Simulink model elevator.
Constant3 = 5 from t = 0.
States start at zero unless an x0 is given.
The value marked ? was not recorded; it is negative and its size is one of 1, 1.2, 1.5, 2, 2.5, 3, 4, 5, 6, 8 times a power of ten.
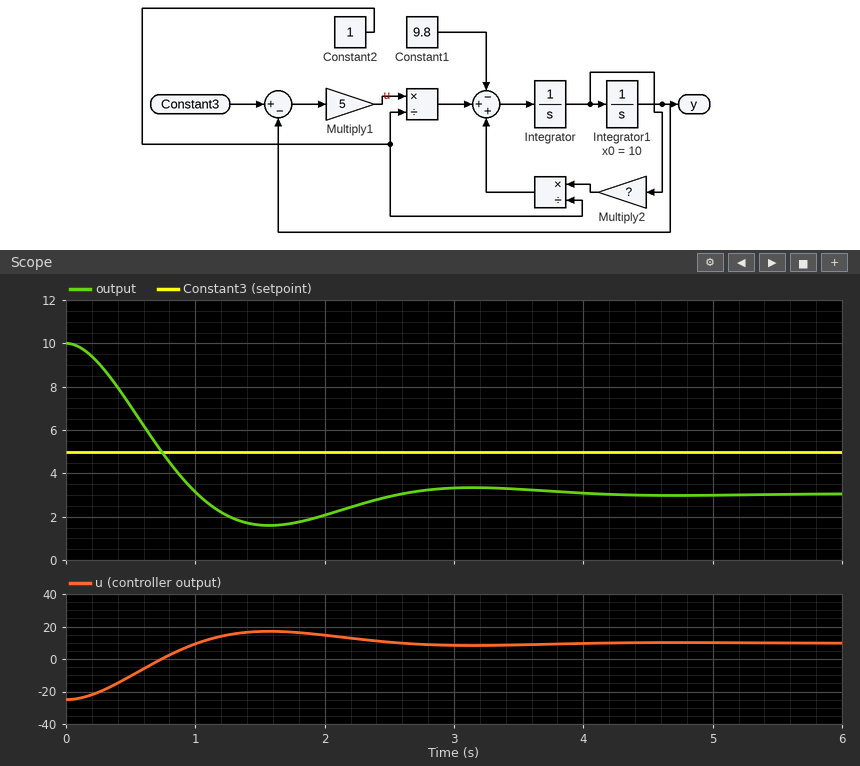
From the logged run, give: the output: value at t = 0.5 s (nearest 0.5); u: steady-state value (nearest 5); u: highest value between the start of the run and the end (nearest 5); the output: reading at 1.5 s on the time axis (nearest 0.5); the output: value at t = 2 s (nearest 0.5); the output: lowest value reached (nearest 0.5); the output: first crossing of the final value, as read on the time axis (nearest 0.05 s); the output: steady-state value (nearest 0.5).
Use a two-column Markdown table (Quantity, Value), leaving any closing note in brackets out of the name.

| Quantity | Value |
|---|---|
| the output: value at t = 0.5 s | 7.0 |
| u: steady-state value | 10 |
| u: highest value between the start of the run and the end | 15 |
| the output: reading at 1.5 s on the time axis | 1.5 |
| the output: value at t = 2 s | 2.0 |
| the output: lowest value reached | 1.5 |
| the output: first crossing of the final value, as read on the time axis | 1.00 s |
| the output: steady-state value | 3.0 |
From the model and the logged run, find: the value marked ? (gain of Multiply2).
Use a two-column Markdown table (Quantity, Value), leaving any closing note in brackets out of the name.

| Quantity | Value |
|---|---|
| the value marked ? | -2 |
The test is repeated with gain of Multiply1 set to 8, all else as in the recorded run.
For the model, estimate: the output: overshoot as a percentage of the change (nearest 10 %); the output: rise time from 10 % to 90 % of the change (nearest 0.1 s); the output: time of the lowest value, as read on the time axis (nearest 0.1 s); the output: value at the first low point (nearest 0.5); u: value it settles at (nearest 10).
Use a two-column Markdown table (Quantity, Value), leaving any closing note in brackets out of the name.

| Quantity | Value |
|---|---|
| the output: overshoot as a percentage of the change | 30 % |
| the output: rise time from 10 % to 90 % of the change | 0.5 s |
| the output: time of the lowest value, as read on the time axis | 1.2 s |
| the output: value at the first low point | 2.0 |
| u: value it settles at | 10 |
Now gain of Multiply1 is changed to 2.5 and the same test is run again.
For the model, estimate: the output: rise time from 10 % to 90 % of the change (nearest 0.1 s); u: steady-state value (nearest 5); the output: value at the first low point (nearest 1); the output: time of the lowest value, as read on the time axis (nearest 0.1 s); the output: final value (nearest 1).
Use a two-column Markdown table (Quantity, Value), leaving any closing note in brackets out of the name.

| Quantity | Value |
|---|---|
| the output: rise time from 10 % to 90 % of the change | 1.2 s |
| u: steady-state value | 10 |
| the output: value at the first low point | 0 |
| the output: time of the lowest value, as read on the time axis | 2.6 s |
| the output: final value | 1 |
